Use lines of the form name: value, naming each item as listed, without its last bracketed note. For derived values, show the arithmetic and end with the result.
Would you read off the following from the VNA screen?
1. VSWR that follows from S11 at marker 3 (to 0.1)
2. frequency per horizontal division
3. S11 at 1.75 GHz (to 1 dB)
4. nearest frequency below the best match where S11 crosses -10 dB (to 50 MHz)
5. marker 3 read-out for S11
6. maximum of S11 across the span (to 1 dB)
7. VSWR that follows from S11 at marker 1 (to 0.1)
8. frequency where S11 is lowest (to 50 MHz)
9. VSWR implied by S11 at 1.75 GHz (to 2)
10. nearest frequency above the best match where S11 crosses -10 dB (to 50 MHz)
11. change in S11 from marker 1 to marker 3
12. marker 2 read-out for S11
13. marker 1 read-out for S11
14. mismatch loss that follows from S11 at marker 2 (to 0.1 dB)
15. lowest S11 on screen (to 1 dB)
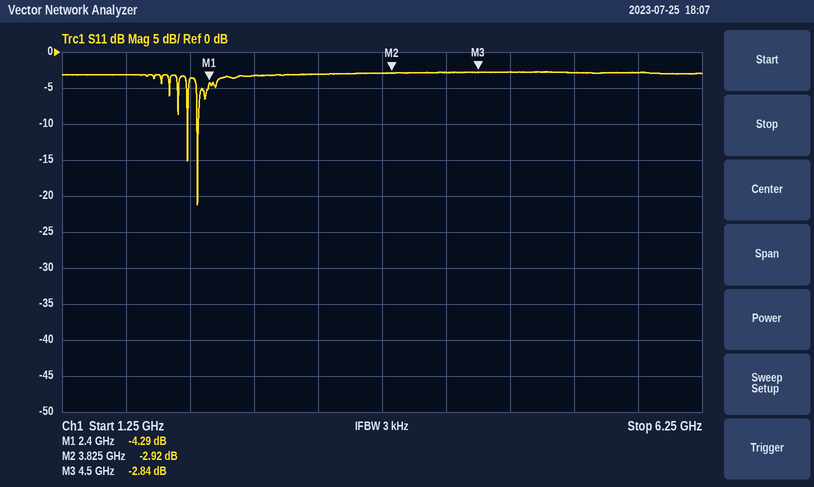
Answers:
VSWR that follows from S11 at marker 3: (1 + 0.7211)/(1 − 0.7211) ≈ 6.2
frequency per horizontal division: 500 MHz
S11 at 1.75 GHz: -3 dB
nearest frequency below the best match where S11 crosses -10 dB: 2.30 GHz
marker 3 read-out for S11: -2.84 dB
maximum of S11 across the span: -3 dB
VSWR that follows from S11 at marker 1: (1 + 0.6102)/(1 − 0.6102) ≈ 4.1
frequency where S11 is lowest: 2.30 GHz
VSWR implied by S11 at 1.75 GHz: |Γ| = 10^(-3/20) = 0.7079; VSWR = (1 + 0.7079)/(1 − 0.7079) ≈ 6
nearest frequency above the best match where S11 crosses -10 dB: 2.30 GHz
change in S11 from marker 1 to marker 3: -2.84 − (-4.29) = 1.45 dB
marker 2 read-out for S11: -2.92 dB
marker 1 read-out for S11: -4.29 dB
mismatch loss that follows from S11 at marker 2: −10 log10(1 − 10^(-2.92/10)) ≈ 3.1 dB
lowest S11 on screen: -21 dB
